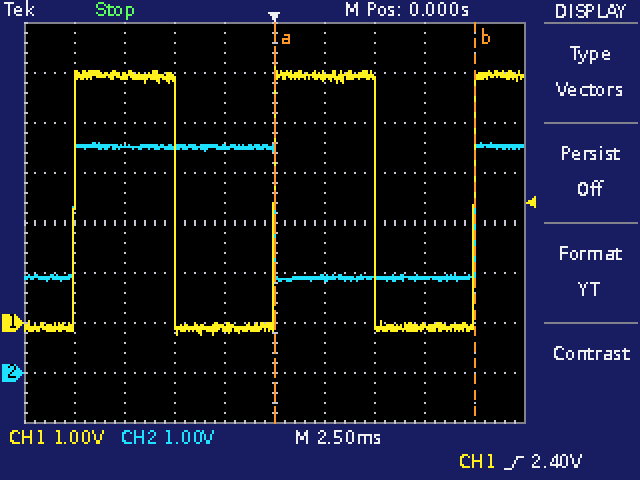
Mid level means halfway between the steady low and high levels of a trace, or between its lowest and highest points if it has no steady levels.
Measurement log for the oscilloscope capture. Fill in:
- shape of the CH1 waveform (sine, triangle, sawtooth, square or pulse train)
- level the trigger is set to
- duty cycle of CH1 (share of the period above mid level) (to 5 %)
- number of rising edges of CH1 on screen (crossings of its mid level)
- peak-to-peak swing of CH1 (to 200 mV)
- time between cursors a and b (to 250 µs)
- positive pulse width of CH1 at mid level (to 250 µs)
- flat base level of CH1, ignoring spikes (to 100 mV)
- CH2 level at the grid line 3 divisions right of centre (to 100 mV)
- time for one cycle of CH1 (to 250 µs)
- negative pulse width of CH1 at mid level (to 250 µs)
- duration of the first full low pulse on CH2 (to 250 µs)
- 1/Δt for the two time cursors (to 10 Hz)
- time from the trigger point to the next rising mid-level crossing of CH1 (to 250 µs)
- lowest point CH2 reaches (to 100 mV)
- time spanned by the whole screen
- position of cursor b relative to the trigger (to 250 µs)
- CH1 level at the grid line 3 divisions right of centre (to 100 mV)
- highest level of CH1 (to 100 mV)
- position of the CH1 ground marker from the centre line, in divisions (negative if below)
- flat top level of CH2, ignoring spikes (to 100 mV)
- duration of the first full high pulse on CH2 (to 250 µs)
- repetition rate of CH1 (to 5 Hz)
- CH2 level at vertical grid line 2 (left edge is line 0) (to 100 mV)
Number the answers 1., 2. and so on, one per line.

1. square
2. 2.40 V
3. 50 %
4. 3
5. 5.4 V
6. 10.00 ms
7. 5.00 ms
8. -100 mV
9. 1.9 V
10. 10.00 ms
11. 5.00 ms
12. 10.00 ms
13. 100 Hz
14. 10.00 ms
15. 1.8 V
16. 25 ms
17. +10.00 ms
18. -100 mV
19. 5.1 V
20. -2.0 div
21. 4.5 V
22. 10.00 ms
23. 100 Hz
24. 4.5 V
